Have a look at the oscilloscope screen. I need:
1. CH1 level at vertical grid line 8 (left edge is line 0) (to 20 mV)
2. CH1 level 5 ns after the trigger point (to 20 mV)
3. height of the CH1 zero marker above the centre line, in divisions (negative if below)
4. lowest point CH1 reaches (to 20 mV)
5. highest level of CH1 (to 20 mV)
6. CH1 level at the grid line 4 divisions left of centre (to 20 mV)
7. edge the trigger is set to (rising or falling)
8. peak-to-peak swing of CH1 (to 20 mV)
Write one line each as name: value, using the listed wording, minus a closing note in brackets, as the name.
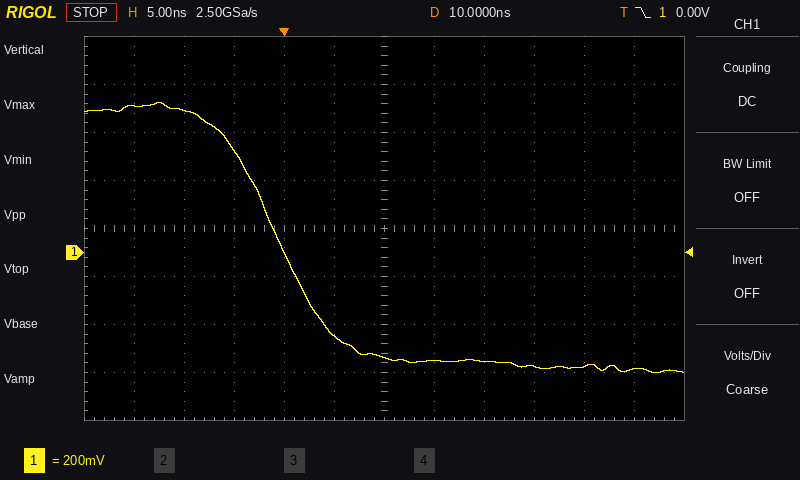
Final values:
CH1 level at vertical grid line 8 (left edge is line 0): -460 mV
CH1 level 5 ns after the trigger point: -340 mV
height of the CH1 zero marker above the centre line, in divisions: -0.5 div
lowest point CH1 reaches: -500 mV
highest level of CH1: 620 mV
CH1 level at the grid line 4 divisions left of centre: 600 mV
edge the trigger is set to: falling
peak-to-peak swing of CH1: 1.12 V
